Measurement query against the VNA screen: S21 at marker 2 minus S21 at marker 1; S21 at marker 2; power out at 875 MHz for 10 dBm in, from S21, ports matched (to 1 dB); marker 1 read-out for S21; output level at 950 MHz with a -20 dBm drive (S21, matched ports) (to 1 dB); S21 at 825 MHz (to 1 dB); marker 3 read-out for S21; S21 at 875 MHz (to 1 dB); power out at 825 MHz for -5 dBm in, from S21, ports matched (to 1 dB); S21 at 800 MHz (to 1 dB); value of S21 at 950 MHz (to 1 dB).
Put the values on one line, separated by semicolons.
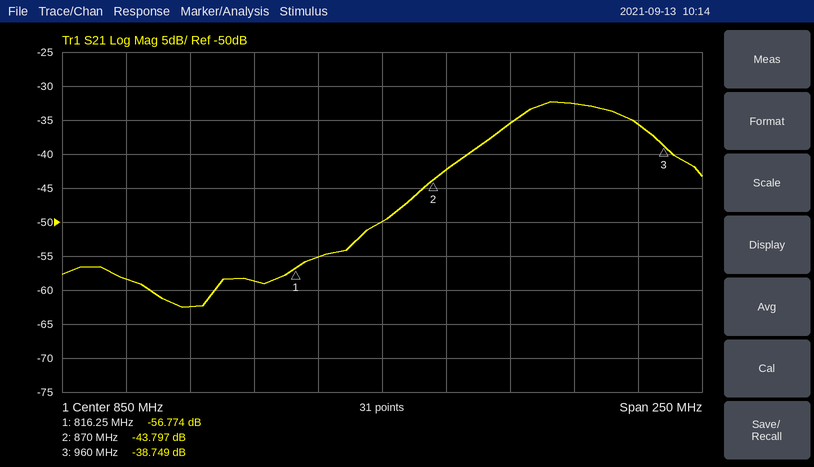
12.977 dB; -43.797 dB; -32 dBm; -56.774 dB; -56 dBm; -55 dB; -38.749 dB; -42 dB; -60 dBm; -59 dB; -36 dB
